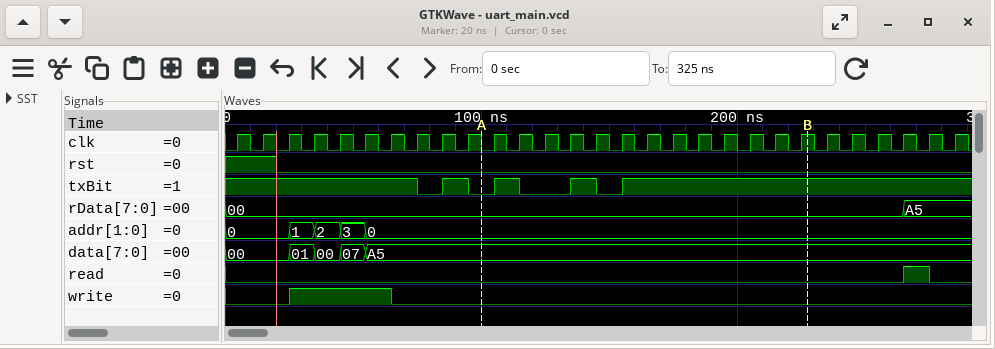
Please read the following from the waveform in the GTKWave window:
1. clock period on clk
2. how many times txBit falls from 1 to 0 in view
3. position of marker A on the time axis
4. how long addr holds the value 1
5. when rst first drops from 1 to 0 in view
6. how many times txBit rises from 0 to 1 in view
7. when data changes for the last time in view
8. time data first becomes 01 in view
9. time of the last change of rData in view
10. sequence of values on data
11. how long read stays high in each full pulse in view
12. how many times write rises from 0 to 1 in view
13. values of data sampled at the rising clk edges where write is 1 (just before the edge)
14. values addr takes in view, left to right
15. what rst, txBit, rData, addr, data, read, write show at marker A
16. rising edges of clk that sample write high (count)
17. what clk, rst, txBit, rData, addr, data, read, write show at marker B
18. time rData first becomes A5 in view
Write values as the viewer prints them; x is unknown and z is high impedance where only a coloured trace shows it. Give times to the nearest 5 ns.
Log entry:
10 ns
4
100 ns
10 ns
20 ns
4
55 ns
25 ns
265 ns
00, 01, 00, 07, A5
10 ns
1
01, 00, 07, A5
0, 1, 2, 3, 0
rst=0, txBit=0, rData=00, addr=0, data=A5, read=0, write=0
4
clk=1, rst=0, txBit=1, rData=00, addr=0, data=A5, read=0, write=0
265 ns
